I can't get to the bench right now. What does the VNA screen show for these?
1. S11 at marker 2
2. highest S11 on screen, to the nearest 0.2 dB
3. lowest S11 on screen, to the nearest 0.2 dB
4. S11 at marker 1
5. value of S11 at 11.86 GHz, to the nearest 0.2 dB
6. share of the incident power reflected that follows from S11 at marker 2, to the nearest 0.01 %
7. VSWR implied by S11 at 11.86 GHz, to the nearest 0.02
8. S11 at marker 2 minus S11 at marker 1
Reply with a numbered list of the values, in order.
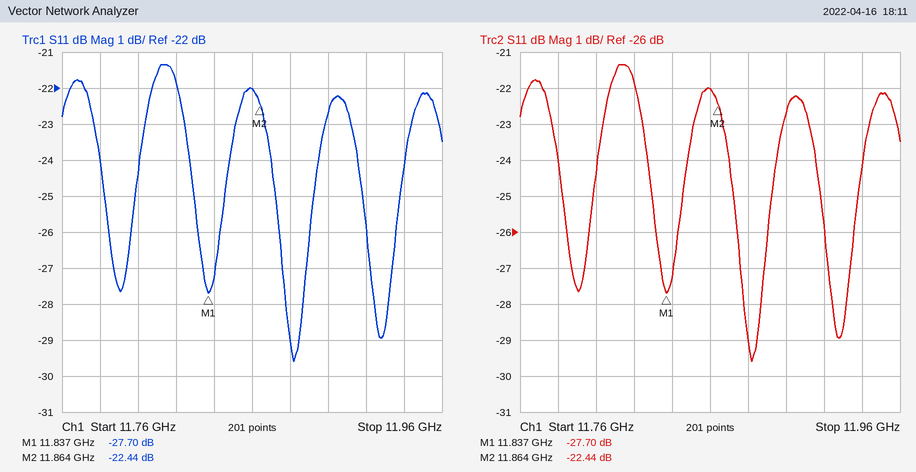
1. -22.44 dB
2. -21.4 dB
3. -29.6 dB
4. -27.70 dB
5. -22.0 dB
6. 0.57 %
7. 1.18
8. 5.26 dB
